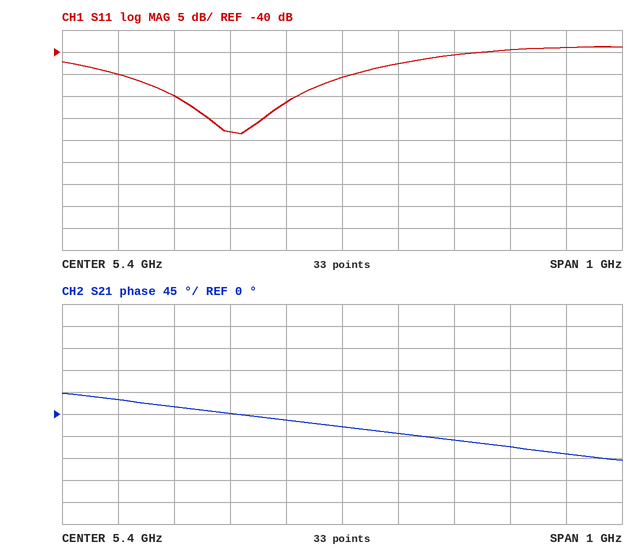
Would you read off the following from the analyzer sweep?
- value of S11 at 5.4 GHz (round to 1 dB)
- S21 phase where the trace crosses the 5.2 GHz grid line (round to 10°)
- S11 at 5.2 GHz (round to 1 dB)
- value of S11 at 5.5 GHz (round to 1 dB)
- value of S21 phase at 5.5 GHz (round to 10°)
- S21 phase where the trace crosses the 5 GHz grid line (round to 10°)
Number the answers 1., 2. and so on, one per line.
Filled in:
1. -46 dB
2. 0°
3. -58 dB
4. -43 dB
5. -40°
6. 30°
